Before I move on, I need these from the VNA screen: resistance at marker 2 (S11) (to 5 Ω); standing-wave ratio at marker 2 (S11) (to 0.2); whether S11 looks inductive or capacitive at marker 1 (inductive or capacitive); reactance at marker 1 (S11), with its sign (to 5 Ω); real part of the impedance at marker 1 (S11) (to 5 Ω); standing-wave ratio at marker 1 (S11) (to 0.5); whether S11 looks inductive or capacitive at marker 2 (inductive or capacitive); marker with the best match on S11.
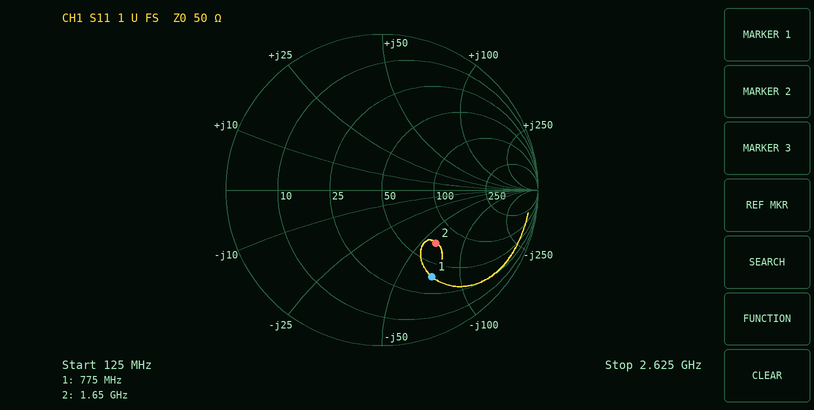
70 Ω
2.8
capacitive
-70 Ω
40 Ω
4.5
capacitive
marker 2
